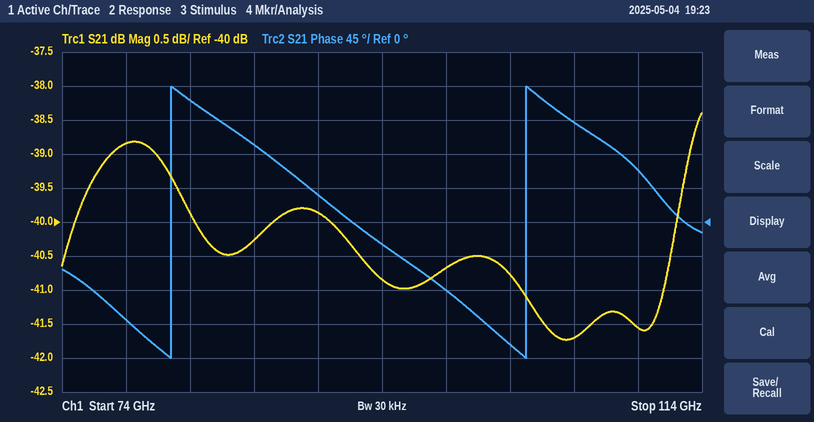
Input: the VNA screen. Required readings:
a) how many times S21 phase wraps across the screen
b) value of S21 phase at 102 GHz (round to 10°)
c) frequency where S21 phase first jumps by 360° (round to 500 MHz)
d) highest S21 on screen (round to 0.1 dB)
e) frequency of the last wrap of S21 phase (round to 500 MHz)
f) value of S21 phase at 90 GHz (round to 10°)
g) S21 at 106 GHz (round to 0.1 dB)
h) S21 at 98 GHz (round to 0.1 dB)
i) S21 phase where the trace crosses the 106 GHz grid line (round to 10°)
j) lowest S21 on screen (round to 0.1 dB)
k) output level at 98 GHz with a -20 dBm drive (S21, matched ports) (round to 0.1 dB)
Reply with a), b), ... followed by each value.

a) 2
b) -160°
c) 81.0 GHz
d) -38.4 dB
e) 103.0 GHz
f) 40°
g) -41.7 dB
h) -40.7 dB
i) 130°
j) -41.7 dB
k) -60.7 dBm
